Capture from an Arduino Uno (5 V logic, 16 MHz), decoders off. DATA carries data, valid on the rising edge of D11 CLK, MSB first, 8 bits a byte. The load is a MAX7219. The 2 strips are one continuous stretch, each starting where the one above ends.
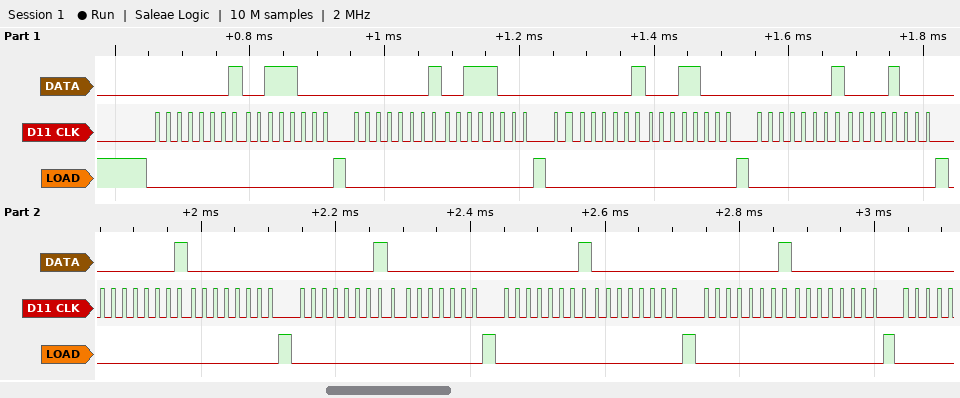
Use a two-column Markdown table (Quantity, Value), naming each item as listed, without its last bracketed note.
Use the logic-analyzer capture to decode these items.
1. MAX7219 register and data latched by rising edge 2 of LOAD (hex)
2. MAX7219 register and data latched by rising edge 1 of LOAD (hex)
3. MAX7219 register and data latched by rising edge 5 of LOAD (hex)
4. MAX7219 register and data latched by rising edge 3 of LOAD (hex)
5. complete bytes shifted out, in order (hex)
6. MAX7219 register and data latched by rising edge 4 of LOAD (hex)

| Quantity | Value |
|---|---|
| MAX7219 register and data latched by rising edge 2 of LOAD | register 0x1, data 0x38 |
| MAX7219 register and data latched by rising edge 1 of LOAD | register 0x1, data 0x38 |
| MAX7219 register and data latched by rising edge 5 of LOAD | register 0x1, data 0x00 |
| MAX7219 register and data latched by rising edge 3 of LOAD | register 0x1, data 0x18 |
| complete bytes shifted out, in order | 0x01 0x38 0x01 0x38 0x01 0x18 0x01 0x08 0x01 0x00 0x01 0x00 0x01 0x00 0x01 0x00 |
| MAX7219 register and data latched by rising edge 4 of LOAD | register 0x1, data 0x08 |
